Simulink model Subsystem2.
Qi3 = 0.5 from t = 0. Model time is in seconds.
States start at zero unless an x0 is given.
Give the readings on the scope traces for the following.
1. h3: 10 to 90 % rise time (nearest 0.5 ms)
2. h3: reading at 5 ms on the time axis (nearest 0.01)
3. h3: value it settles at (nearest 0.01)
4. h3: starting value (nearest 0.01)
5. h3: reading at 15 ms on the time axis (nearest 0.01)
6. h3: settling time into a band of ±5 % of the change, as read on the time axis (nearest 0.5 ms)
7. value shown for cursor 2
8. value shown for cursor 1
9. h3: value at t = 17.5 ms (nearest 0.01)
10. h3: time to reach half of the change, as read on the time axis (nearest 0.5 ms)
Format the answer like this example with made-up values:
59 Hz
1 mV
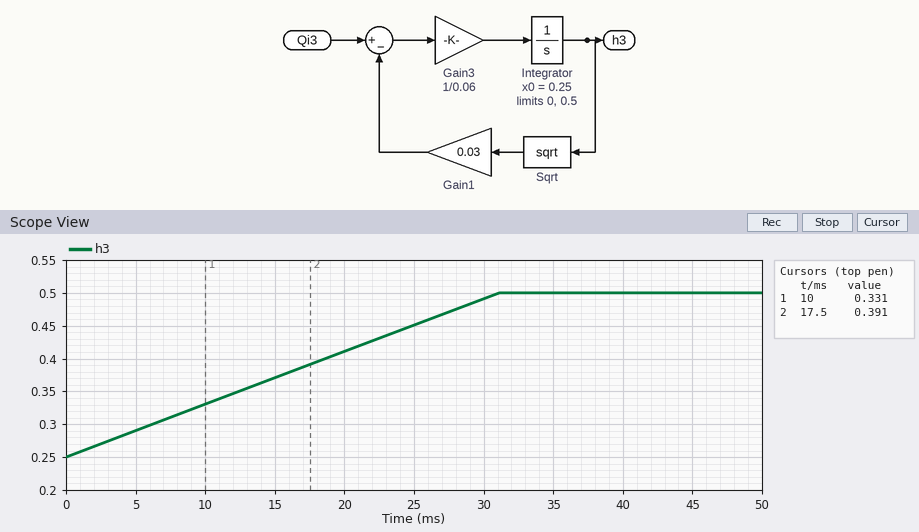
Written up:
25.0 ms
0.29
0.50
0.25
0.37
29.5 ms
0.391
0.331
0.39
15.5 ms
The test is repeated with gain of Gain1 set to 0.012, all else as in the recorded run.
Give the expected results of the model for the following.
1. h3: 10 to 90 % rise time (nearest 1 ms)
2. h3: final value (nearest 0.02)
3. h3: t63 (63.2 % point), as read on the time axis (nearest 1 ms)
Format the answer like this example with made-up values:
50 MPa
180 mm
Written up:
24 ms
0.50
19 ms
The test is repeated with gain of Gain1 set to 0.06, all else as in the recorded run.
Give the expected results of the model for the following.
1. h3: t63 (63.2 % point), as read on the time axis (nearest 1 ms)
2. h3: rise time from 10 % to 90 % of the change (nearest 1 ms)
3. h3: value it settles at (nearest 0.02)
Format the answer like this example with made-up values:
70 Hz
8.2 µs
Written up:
20 ms
26 ms
0.50
